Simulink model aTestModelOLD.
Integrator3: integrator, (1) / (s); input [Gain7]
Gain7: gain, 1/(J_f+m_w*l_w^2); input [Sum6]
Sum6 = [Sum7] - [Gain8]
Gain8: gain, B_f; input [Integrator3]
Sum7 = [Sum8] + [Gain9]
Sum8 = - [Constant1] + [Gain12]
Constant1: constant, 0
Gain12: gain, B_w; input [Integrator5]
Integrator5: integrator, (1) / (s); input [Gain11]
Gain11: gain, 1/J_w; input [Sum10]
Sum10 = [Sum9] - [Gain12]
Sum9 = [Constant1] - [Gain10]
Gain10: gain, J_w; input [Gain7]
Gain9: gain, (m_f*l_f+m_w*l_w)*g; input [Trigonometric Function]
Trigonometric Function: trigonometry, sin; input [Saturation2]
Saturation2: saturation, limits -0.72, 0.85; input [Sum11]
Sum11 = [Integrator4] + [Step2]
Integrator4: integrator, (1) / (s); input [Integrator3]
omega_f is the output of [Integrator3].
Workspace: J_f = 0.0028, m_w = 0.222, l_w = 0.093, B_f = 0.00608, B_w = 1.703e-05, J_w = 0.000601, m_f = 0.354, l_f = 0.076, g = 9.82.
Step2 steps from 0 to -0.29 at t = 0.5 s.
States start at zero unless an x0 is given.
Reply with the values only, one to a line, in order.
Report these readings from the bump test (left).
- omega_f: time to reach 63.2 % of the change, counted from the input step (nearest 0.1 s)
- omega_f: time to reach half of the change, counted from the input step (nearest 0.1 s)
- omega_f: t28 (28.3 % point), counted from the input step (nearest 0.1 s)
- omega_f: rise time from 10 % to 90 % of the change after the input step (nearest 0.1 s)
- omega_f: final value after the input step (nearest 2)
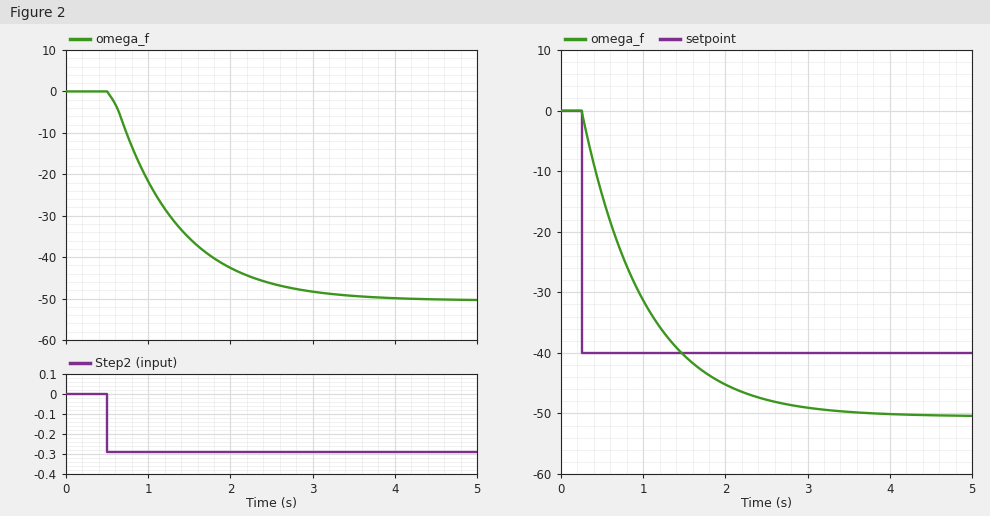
0.8 s
0.6 s
0.3 s
1.7 s
-50
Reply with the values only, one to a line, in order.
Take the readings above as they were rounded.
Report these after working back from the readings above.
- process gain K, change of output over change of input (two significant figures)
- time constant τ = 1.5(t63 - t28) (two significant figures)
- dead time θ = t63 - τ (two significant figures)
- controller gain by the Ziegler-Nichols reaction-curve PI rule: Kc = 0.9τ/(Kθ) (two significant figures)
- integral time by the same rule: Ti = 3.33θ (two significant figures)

170
0.75 s
0.050 s
0.079
0.17 s
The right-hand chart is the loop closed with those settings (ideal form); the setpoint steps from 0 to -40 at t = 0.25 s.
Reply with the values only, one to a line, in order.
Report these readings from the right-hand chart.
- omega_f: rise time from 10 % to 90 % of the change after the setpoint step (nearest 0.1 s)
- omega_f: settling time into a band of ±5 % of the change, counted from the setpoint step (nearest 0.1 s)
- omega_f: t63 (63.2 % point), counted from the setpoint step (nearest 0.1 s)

1.7 s
2.3 s
0.8 s
